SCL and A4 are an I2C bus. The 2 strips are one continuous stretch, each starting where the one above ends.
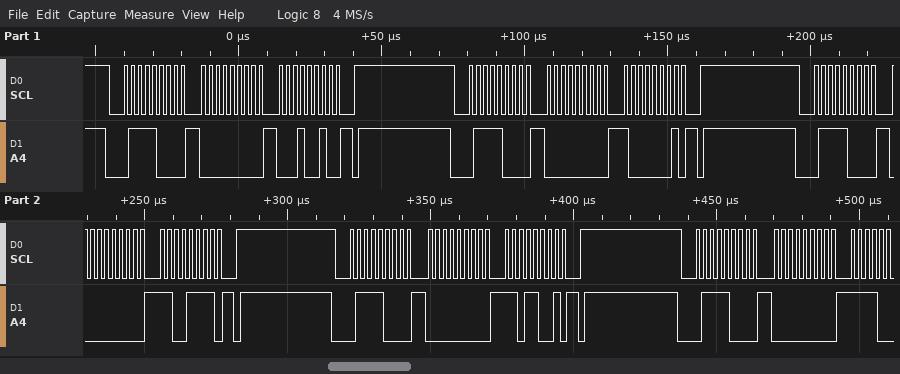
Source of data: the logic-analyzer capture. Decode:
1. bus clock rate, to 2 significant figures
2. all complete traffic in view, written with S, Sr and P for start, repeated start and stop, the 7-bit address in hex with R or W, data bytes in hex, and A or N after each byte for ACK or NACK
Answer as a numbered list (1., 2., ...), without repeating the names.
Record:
1. 400 kHz
2. S 3CW A 00 A 12 A P S 3CW A 00 A 81 A P S 3CW A 00 A CF A P S 3CW A 00 A D9 A P S 3CW A 00 A
